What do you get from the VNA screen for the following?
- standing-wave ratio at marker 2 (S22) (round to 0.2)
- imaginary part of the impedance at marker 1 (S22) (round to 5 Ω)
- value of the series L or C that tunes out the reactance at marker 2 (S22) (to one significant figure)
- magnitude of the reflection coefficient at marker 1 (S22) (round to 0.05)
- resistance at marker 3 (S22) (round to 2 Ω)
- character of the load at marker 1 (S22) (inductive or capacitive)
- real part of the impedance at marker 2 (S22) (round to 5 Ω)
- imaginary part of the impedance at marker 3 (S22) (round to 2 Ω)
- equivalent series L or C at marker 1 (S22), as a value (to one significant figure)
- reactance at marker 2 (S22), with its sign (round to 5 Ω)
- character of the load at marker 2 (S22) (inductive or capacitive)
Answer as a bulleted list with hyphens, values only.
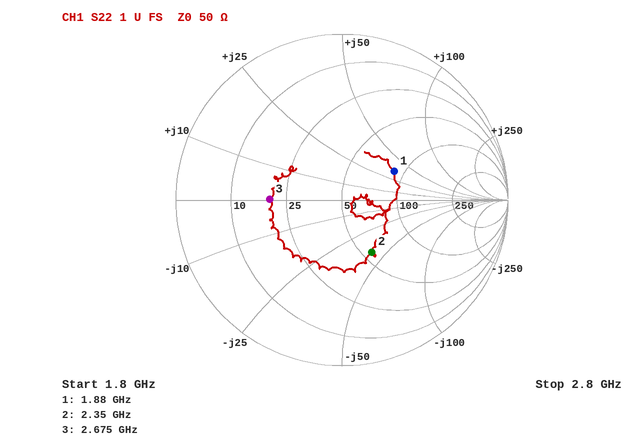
- 2.2
- +35 Ω
- 3 nH
- 0.35
- 20 Ω
- inductive
- 55 Ω
- 0 Ω
- 3 nH
- -40 Ω
- capacitive
